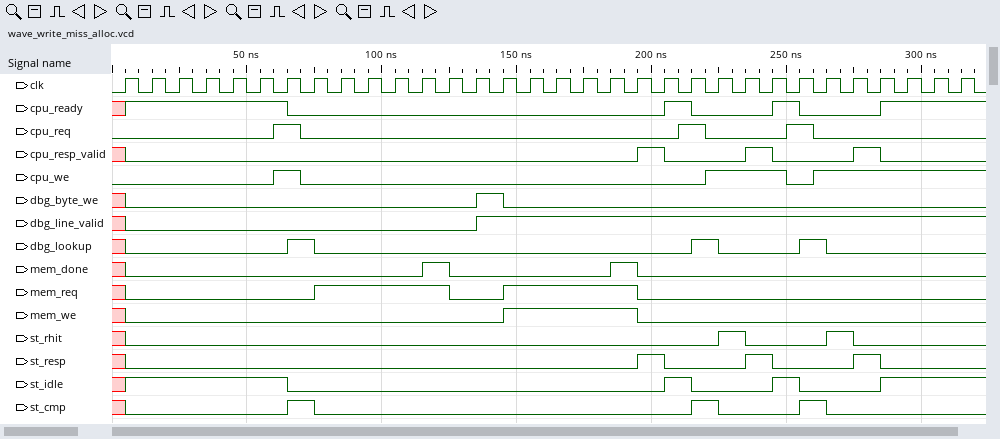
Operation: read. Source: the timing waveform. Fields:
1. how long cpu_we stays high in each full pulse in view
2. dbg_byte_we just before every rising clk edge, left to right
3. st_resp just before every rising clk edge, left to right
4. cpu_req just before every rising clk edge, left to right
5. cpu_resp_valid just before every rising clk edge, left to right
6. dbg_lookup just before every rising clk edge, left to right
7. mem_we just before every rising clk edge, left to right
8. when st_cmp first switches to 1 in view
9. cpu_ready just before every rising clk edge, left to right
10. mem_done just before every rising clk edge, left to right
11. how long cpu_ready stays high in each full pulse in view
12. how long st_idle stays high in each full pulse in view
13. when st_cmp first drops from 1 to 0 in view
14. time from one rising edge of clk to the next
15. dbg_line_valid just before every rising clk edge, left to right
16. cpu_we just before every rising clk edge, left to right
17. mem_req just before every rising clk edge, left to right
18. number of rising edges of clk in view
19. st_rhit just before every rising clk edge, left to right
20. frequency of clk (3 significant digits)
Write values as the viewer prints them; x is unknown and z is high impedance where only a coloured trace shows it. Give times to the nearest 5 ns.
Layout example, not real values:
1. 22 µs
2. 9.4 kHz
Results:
1. 10 ns, 30 ns
2. x 0 0 0 0 0 0 0 0 0 0 0 0 0 1 0 0 0 0 0 0 0 0 0 0 0 0 0 0 0 0 0
3. x 0 0 0 0 0 0 0 0 0 0 0 0 0 0 0 0 0 0 0 1 0 0 0 1 0 0 0 1 0 0 0
4. 0 0 0 0 0 0 1 0 0 0 0 0 0 0 0 0 0 0 0 0 0 1 0 0 0 1 0 0 0 0 0 0
5. x 0 0 0 0 0 0 0 0 0 0 0 0 0 0 0 0 0 0 0 1 0 0 0 1 0 0 0 1 0 0 0
6. x 0 0 0 0 0 0 1 0 0 0 0 0 0 0 0 0 0 0 0 0 0 1 0 0 0 1 0 0 0 0 0
7. x 0 0 0 0 0 0 0 0 0 0 0 0 0 0 1 1 1 1 1 0 0 0 0 0 0 0 0 0 0 0 0
8. 65 ns
9. x 1 1 1 1 1 1 0 0 0 0 0 0 0 0 0 0 0 0 0 0 1 0 0 0 1 0 0 0 1 1 1
10. x 0 0 0 0 0 0 0 0 0 0 0 1 0 0 0 0 0 0 1 0 0 0 0 0 0 0 0 0 0 0 0
11. 10 ns, 10 ns
12. 10 ns, 10 ns
13. 75 ns
14. 10 ns
15. x 0 0 0 0 0 0 0 0 0 0 0 0 0 1 1 1 1 1 1 1 1 1 1 1 1 1 1 1 1 1 1
16. 0 0 0 0 0 0 1 0 0 0 0 0 0 0 0 0 0 0 0 0 0 0 1 1 1 0 1 1 1 1 1 1
17. x 0 0 0 0 0 0 0 1 1 1 1 1 0 0 1 1 1 1 1 0 0 0 0 0 0 0 0 0 0 0 0
18. 32
19. x 0 0 0 0 0 0 0 0 0 0 0 0 0 0 0 0 0 0 0 0 0 0 1 0 0 0 1 0 0 0 0
20. 100 MHz
